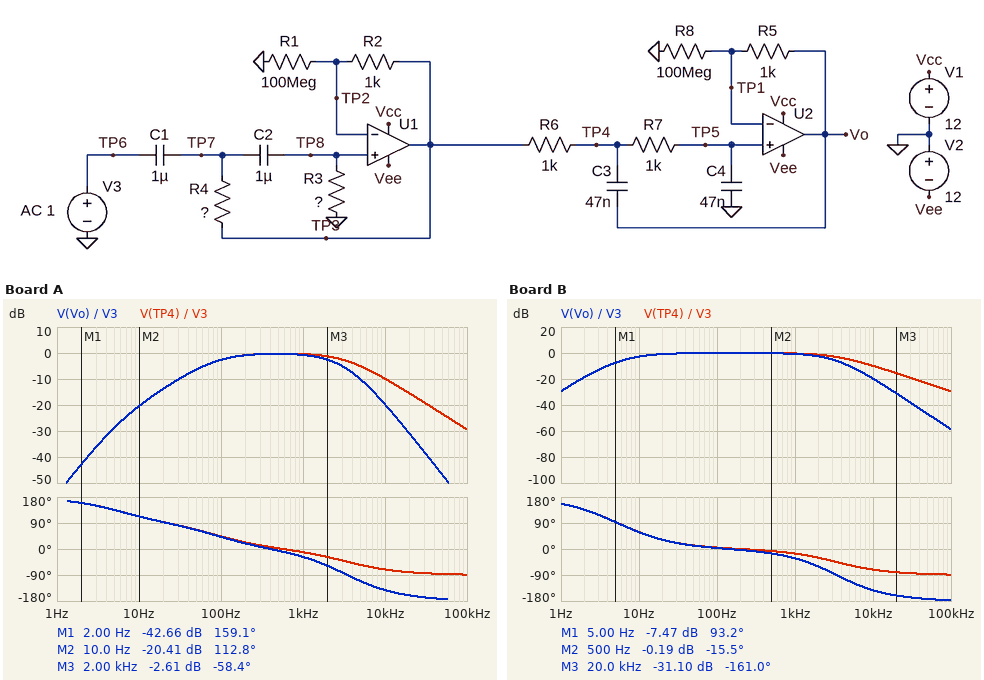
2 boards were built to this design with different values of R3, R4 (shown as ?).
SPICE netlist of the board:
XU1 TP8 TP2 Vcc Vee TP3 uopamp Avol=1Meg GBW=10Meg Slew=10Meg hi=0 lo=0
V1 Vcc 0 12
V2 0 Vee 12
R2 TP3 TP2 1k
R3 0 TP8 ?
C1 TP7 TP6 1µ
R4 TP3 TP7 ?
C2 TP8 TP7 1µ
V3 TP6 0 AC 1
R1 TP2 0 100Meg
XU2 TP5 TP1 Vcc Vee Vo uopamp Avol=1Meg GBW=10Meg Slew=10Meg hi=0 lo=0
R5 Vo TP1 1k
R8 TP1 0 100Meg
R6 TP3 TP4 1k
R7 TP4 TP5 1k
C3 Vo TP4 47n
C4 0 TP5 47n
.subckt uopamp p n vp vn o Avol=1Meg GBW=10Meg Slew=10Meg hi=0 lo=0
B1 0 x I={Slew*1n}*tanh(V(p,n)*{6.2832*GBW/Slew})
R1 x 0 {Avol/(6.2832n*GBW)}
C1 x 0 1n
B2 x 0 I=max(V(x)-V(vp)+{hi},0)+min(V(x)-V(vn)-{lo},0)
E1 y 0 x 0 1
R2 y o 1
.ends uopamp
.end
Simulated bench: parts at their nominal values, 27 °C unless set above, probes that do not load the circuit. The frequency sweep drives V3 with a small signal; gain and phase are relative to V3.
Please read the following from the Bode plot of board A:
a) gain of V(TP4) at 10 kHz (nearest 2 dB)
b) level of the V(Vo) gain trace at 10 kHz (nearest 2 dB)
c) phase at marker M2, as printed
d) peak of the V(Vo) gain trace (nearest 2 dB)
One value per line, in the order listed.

-10 dB
-20 dB
112.8 deg
0 dB
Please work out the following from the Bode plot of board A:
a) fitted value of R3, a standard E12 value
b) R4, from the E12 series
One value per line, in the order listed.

3.3 kΩ
15 kΩ
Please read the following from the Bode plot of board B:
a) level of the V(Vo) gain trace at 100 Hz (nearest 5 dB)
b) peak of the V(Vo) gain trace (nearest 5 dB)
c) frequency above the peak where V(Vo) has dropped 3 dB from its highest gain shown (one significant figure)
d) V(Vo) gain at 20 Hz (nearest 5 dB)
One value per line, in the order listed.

0 dB
0 dB
2 kHz
0 dB
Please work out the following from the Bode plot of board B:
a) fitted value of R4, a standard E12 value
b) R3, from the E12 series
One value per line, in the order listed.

33 kΩ
27 kΩ
